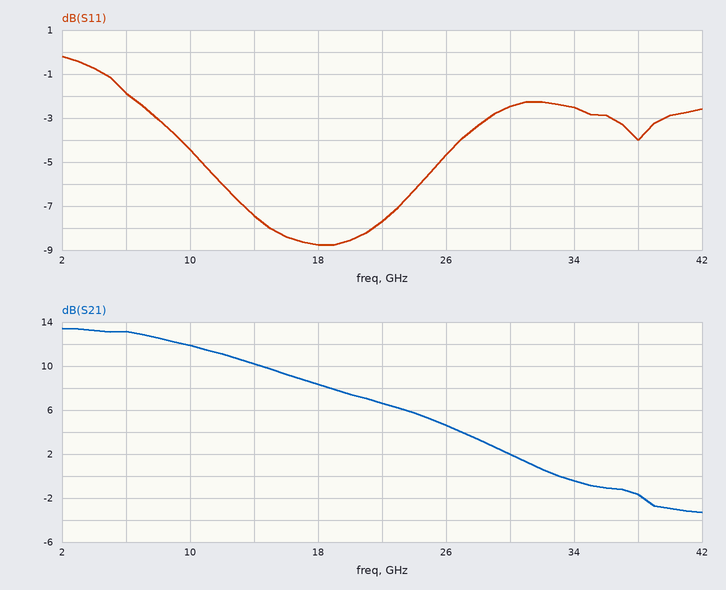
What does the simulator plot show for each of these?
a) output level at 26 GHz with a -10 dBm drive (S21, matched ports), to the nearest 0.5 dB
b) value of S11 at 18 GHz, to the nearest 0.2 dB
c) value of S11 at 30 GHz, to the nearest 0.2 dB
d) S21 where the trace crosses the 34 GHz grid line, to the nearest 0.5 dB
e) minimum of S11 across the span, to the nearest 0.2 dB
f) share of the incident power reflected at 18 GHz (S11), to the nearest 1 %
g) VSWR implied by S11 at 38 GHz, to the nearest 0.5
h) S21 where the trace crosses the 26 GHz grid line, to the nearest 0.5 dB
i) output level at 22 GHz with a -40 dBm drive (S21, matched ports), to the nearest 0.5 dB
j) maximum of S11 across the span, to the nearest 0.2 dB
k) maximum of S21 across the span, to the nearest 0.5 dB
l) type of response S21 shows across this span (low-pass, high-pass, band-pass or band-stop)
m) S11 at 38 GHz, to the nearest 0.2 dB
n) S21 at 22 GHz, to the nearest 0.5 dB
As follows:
-5.5 dBm
-8.8 dB
-2.4 dB
-0.5 dB
-8.8 dB
13 %
4.5
4.5 dB
-33.5 dBm
-0.2 dB
13.5 dB
low-pass
-4.0 dB
6.5 dB
